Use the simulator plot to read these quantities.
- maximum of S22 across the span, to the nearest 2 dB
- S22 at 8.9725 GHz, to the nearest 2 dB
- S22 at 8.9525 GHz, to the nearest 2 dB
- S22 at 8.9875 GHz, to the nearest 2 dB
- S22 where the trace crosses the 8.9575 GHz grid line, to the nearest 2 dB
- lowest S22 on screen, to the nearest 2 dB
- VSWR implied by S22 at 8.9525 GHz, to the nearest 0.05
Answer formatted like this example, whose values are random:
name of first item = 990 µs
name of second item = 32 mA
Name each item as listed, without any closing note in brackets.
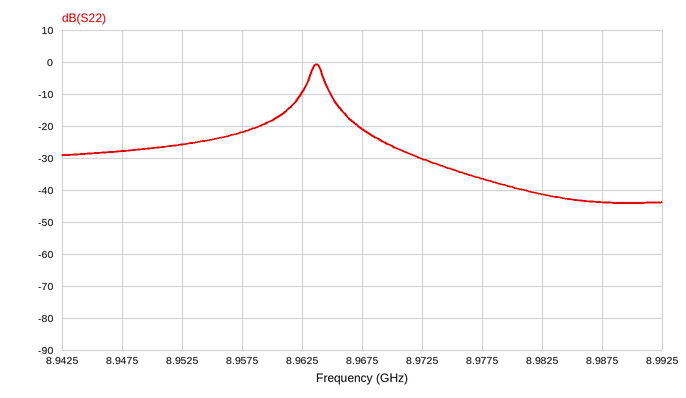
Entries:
maximum of S22 across the span, to the nearest 2 dB = 0 dB
S22 at 8.9725 GHz, to the nearest 2 dB = -30 dB
S22 at 8.9525 GHz, to the nearest 2 dB = -26 dB
S22 at 8.9875 GHz, to the nearest 2 dB = -44 dB
S22 where the trace crosses the 8.9575 GHz grid line, to the nearest 2 dB = -22 dB
lowest S22 on screen, to the nearest 2 dB = -44 dB
VSWR implied by S22 at 8.9525 GHz, to the nearest 0.05 = 1.10
